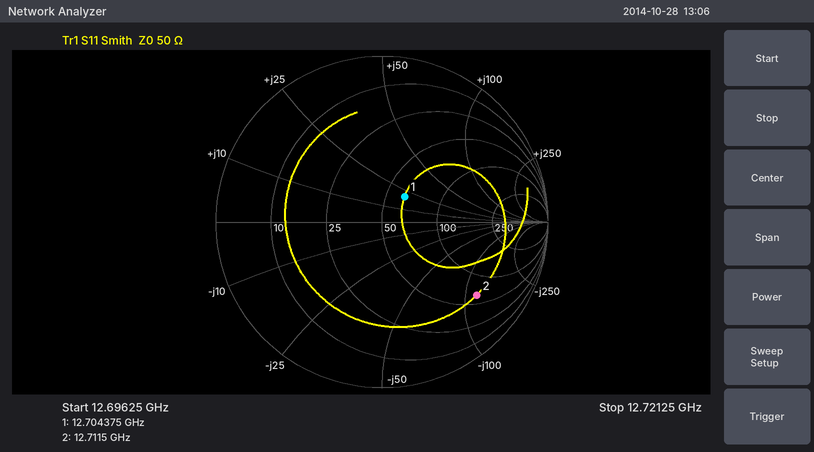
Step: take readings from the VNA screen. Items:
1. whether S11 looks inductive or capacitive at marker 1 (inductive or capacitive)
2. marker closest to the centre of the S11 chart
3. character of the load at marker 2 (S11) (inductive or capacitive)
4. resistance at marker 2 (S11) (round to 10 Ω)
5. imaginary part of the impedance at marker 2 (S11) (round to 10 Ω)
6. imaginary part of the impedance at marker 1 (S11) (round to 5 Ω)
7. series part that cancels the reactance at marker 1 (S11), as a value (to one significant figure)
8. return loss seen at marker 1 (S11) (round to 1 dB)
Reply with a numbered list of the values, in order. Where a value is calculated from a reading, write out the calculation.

1. inductive
2. marker 1
3. capacitive
4. 60 Ω
5. -120 Ω
6. +20 Ω
7. C = 1/(2π × 12.704375 GHz × 20 Ω) ≈ 626 fF, so 600 fF to one significant figure
8. 14 dB
